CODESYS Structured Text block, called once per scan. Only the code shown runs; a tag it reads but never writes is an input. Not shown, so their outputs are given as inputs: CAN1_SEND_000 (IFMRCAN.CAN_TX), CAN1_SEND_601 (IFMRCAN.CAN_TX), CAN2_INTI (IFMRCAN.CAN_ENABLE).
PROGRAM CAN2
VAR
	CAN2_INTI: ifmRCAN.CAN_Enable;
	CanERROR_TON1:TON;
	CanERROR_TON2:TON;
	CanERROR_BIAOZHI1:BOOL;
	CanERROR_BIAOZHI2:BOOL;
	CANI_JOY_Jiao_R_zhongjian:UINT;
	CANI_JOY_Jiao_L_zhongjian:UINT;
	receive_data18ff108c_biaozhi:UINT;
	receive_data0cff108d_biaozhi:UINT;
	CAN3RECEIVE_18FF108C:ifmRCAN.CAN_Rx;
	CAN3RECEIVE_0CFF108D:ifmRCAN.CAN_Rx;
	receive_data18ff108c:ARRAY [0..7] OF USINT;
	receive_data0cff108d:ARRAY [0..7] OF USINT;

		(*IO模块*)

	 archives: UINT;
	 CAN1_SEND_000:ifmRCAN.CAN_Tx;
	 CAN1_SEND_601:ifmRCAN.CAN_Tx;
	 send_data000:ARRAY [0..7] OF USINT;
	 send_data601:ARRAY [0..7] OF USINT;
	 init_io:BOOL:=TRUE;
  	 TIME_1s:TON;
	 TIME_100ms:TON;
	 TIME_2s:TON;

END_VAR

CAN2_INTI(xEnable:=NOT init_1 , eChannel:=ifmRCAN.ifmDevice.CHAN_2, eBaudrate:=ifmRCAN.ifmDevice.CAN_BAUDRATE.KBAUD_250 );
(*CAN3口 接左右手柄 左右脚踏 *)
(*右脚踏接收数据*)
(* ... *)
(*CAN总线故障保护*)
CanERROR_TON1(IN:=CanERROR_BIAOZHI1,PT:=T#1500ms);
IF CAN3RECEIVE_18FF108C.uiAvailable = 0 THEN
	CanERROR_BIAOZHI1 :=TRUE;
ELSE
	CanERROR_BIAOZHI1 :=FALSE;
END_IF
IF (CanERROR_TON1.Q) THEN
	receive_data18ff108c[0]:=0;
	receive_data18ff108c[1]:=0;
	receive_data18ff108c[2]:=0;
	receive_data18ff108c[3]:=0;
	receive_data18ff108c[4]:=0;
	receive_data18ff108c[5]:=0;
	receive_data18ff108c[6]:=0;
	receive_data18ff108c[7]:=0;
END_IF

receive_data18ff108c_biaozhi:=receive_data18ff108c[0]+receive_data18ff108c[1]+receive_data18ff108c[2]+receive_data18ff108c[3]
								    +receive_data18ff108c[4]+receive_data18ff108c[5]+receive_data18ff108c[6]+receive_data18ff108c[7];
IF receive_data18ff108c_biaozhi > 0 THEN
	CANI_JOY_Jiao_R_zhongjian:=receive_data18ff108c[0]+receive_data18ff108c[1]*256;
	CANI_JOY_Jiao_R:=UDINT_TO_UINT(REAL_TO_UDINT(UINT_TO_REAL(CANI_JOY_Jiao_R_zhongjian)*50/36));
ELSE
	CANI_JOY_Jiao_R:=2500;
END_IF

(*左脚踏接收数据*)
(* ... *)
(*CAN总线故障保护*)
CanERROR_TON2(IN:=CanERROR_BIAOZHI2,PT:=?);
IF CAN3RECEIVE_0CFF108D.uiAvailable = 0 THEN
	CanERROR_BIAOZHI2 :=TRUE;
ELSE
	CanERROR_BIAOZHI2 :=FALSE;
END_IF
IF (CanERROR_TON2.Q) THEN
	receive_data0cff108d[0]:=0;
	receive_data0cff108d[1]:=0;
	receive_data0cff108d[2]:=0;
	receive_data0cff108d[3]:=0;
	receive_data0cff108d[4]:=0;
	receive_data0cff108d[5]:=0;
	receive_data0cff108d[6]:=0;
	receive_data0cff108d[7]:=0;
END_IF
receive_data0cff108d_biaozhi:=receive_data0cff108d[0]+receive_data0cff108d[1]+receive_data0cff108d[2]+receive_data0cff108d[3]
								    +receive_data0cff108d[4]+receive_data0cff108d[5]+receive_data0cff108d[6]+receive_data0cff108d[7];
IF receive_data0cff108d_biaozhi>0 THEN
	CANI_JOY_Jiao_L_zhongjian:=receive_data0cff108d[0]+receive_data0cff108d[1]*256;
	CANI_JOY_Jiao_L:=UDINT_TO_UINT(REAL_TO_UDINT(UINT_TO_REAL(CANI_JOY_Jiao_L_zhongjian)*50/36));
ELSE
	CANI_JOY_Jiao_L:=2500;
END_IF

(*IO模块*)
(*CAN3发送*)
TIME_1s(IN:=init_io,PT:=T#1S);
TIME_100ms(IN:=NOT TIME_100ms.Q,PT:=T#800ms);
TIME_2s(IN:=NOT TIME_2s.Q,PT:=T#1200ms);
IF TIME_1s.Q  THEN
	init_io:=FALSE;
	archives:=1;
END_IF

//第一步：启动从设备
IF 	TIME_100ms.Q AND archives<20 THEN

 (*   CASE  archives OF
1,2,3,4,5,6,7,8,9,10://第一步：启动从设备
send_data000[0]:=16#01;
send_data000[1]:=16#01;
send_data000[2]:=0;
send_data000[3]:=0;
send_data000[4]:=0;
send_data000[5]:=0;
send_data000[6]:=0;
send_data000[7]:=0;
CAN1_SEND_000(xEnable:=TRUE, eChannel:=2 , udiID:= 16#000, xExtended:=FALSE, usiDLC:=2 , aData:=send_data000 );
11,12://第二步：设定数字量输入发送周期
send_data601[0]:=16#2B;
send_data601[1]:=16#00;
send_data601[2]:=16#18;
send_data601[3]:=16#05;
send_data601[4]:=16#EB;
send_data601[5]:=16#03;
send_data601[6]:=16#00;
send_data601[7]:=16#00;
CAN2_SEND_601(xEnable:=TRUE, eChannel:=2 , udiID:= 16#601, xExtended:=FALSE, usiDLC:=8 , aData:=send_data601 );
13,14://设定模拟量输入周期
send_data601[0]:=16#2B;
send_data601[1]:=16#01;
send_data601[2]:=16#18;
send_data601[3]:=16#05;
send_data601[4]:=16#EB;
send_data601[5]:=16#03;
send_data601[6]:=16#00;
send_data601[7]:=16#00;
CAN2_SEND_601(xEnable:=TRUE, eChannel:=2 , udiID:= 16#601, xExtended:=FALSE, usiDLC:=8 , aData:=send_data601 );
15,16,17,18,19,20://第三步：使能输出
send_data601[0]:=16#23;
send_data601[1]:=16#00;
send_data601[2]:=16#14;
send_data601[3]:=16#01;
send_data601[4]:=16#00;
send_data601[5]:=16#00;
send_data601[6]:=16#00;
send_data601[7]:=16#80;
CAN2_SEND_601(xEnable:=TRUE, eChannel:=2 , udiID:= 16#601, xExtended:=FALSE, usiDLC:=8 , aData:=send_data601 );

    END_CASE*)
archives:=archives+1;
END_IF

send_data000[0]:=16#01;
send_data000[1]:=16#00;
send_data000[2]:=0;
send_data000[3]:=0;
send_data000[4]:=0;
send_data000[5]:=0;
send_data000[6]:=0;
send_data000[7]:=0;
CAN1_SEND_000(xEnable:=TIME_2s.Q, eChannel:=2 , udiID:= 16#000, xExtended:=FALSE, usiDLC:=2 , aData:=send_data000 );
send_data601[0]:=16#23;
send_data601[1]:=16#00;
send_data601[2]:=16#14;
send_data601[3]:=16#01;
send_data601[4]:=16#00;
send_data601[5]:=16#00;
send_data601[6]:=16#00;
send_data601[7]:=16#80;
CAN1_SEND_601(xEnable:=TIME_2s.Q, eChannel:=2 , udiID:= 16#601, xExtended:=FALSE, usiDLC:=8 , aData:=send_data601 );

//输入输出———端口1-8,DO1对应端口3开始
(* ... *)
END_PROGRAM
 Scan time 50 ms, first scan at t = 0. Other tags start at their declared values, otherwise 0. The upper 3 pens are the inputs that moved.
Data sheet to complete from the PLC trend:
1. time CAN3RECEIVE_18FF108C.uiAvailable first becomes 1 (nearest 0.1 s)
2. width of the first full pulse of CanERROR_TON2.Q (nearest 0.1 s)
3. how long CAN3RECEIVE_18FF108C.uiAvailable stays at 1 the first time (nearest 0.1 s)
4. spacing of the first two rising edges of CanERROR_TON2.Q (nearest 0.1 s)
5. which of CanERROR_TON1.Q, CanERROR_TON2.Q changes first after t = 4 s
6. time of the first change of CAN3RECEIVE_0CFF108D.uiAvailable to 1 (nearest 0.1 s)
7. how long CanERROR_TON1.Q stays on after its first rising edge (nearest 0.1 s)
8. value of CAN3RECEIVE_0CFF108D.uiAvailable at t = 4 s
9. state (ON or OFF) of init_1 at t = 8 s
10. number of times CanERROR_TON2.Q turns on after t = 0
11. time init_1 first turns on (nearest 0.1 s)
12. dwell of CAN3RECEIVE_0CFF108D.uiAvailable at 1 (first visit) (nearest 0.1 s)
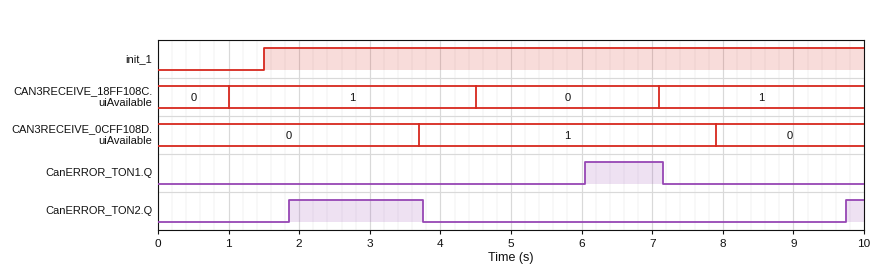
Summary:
1.0 s
1.9 s
3.5 s
7.9 s
CanERROR_TON1.Q
3.7 s
1.1 s
1
ON
2
1.5 s
4.2 s
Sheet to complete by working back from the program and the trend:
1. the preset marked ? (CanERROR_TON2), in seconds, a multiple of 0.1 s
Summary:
1.8 s
